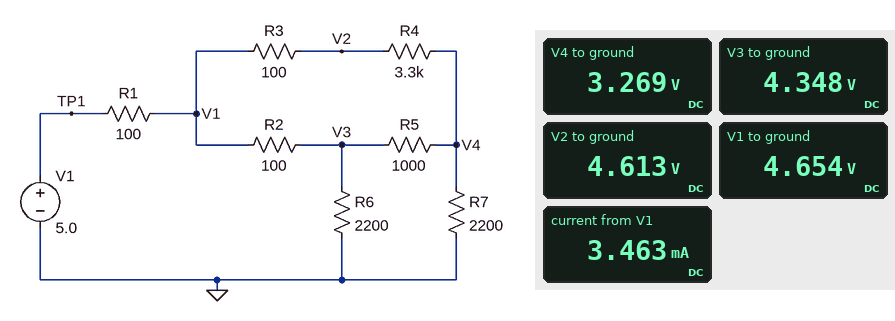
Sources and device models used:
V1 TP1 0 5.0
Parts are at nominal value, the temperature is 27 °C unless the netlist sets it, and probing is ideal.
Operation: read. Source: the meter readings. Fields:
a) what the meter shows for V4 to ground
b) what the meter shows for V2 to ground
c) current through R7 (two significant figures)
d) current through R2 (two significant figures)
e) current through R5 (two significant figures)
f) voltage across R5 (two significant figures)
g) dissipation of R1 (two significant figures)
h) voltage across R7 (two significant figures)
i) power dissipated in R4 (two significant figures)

3.269 V
4.613 V
1.5 mA
3.1 mA
1.1 mA
1.1 V
1.2 mW
3.3 V
550 µW
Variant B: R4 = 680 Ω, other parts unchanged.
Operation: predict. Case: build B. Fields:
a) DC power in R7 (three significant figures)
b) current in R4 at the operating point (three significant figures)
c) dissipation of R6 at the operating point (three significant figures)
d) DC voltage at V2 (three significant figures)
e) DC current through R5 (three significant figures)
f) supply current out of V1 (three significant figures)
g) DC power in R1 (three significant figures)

6.45 mW
1.11 mA
8.68 mW
4.52 V
605 µA
3.70 mA
1.37 mW
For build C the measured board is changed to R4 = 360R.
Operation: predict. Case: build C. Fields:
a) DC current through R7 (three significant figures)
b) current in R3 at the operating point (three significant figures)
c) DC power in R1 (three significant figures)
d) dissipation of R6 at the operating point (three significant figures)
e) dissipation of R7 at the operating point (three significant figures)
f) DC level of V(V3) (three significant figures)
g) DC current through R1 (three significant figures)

1.81 mA
1.40 mA
1.44 mW
8.72 mW
7.18 mW
4.38 V
3.80 mA
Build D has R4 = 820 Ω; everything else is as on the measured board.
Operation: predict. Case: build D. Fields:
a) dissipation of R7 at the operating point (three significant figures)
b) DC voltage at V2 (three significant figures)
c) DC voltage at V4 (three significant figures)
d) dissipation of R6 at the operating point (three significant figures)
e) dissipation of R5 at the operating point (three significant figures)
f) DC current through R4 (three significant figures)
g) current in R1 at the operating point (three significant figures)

6.22 mW
4.53 V
3.70 V
8.67 mW
446 µW
1.01 mA
3.67 mA
